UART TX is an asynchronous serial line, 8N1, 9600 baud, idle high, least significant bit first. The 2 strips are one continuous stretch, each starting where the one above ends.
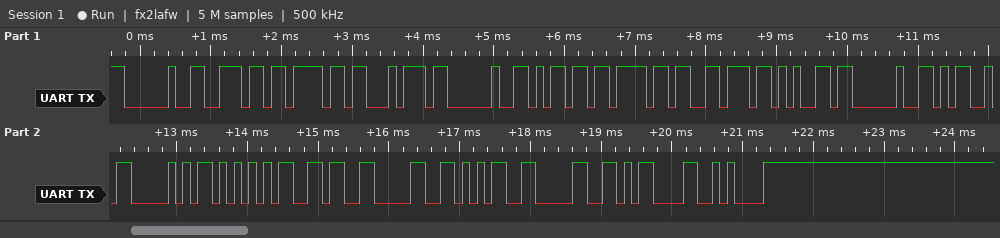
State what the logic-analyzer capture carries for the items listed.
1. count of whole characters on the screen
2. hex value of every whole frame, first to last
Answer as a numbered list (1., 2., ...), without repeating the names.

1. 19
2. 0x20 0x6E 0x6F 0x74 0x20 0x6D 0x6F 0x76 0x65 0x20 0x4D 0x50 0x55 0x36 0x30 0x35 0x30 0x0D 0x0A
